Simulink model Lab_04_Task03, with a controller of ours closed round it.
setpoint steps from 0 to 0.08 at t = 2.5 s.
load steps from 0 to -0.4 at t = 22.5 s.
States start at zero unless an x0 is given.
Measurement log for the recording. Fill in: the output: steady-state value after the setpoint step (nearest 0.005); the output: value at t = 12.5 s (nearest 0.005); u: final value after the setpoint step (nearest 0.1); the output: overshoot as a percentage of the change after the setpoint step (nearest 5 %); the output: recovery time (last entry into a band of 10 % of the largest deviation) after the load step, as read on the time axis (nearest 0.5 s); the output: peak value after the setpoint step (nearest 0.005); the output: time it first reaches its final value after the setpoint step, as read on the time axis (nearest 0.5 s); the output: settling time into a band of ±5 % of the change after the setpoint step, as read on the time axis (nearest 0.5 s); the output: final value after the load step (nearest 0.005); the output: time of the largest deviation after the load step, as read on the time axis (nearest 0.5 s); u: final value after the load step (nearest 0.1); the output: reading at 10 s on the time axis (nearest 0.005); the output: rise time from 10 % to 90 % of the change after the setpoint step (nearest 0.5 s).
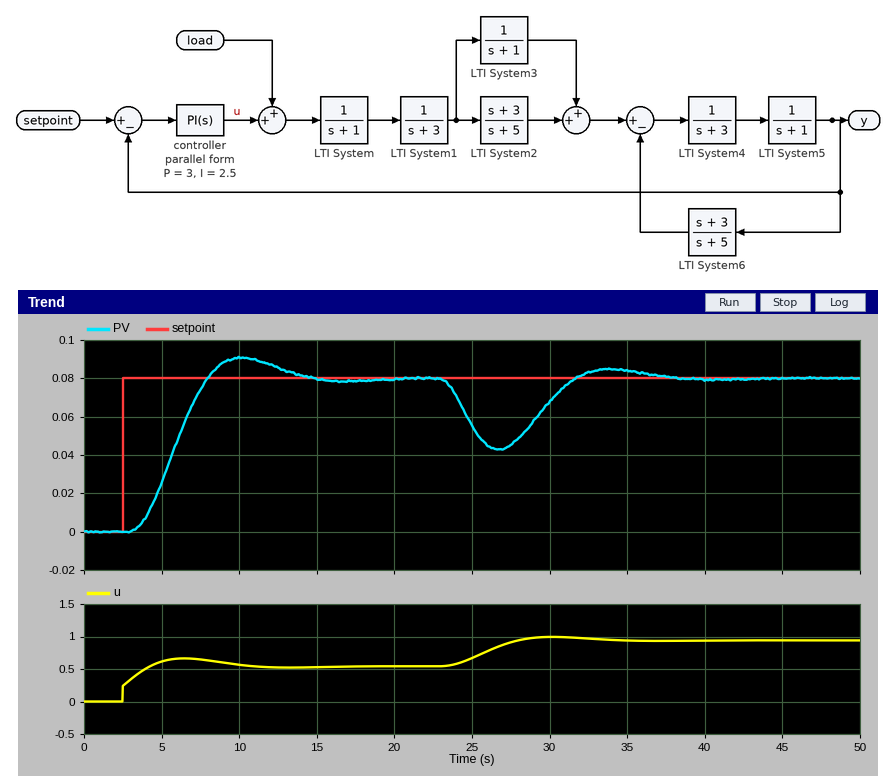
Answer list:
0.080
0.085
0.5
15 %
35.5 s
0.090
8.0 s
13.0 s
0.080
26.5 s
0.9
0.090
3.5 s
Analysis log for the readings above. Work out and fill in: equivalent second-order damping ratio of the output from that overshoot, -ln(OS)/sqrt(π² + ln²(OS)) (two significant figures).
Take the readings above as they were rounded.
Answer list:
0.52
